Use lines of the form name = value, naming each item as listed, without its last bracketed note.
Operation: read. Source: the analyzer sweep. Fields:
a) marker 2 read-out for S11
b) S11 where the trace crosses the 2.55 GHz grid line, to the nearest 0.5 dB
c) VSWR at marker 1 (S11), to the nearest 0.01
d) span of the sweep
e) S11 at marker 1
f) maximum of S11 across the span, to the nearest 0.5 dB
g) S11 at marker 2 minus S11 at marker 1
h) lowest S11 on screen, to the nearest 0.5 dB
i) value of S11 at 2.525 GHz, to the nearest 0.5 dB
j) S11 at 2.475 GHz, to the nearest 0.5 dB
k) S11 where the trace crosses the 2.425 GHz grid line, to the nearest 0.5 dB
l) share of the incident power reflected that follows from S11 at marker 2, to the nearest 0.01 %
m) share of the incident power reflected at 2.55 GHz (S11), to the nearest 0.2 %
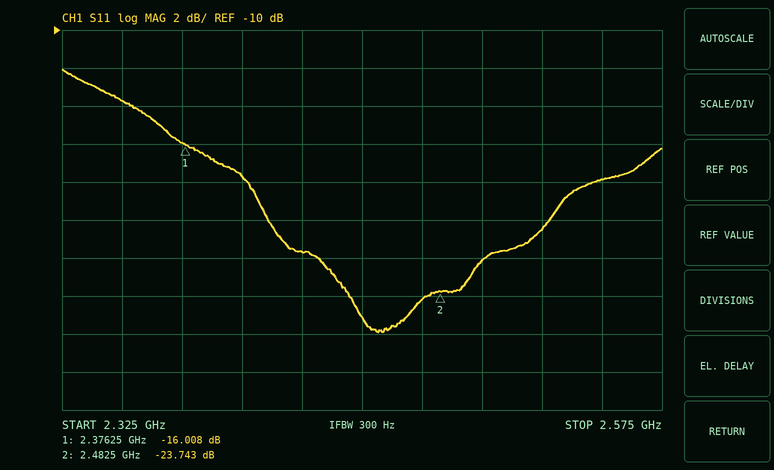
marker 2 read-out for S11 = -23.743 dB
S11 where the trace crosses the 2.55 GHz grid line, to the nearest 0.5 dB = -18.0 dB
VSWR at marker 1 (S11), to the nearest 0.01 = 1.38
span of the sweep = 250 MHz
S11 at marker 1 = -16.008 dB
maximum of S11 across the span, to the nearest 0.5 dB = -12.0 dB
S11 at marker 2 minus S11 at marker 1 = -7.735 dB
lowest S11 on screen, to the nearest 0.5 dB = -26.0 dB
value of S11 at 2.525 GHz, to the nearest 0.5 dB = -20.5 dB
S11 at 2.475 GHz, to the nearest 0.5 dB = -24.0 dB
S11 where the trace crosses the 2.425 GHz grid line, to the nearest 0.5 dB = -21.5 dB
share of the incident power reflected that follows from S11 at marker 2, to the nearest 0.01 % = 0.42 %
share of the incident power reflected at 2.55 GHz (S11), to the nearest 0.2 % = 1.6 %
